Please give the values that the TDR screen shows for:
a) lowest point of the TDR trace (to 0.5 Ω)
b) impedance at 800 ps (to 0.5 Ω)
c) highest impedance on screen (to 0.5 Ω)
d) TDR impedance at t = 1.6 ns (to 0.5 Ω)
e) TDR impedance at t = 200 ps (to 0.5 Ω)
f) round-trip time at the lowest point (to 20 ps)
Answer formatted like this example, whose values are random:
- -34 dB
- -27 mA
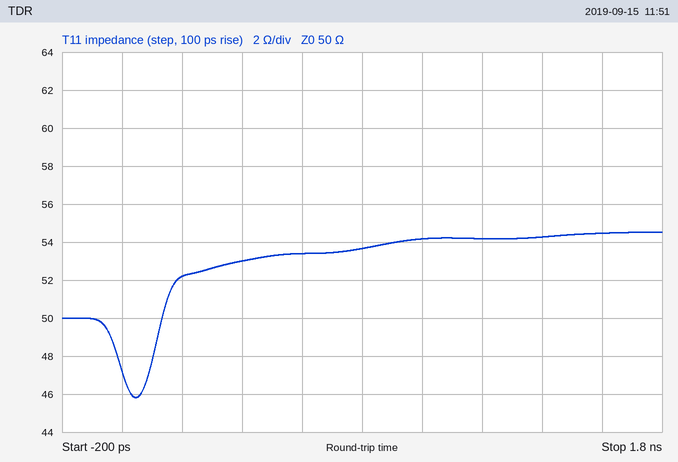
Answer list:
- 46.0 Ω
- 53.5 Ω
- 54.5 Ω
- 54.5 Ω
- 52.0 Ω
- 40 ps
